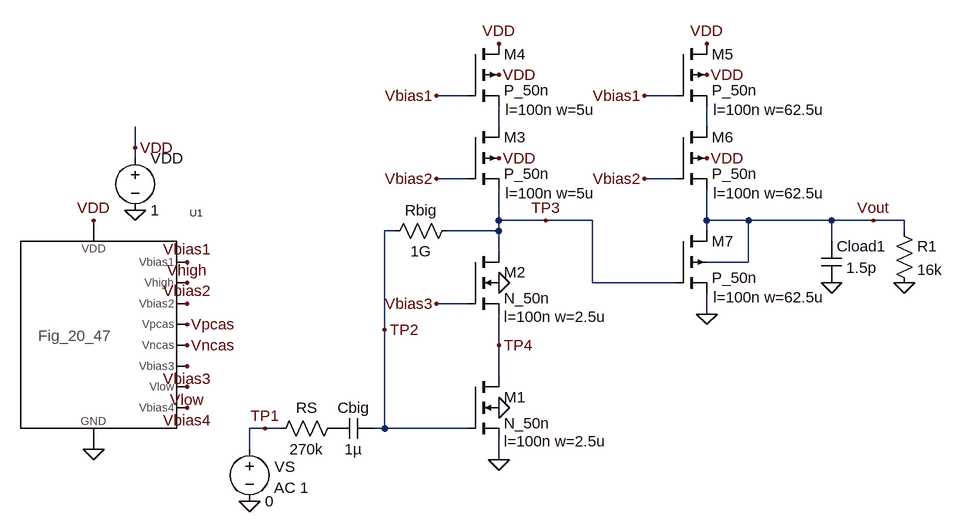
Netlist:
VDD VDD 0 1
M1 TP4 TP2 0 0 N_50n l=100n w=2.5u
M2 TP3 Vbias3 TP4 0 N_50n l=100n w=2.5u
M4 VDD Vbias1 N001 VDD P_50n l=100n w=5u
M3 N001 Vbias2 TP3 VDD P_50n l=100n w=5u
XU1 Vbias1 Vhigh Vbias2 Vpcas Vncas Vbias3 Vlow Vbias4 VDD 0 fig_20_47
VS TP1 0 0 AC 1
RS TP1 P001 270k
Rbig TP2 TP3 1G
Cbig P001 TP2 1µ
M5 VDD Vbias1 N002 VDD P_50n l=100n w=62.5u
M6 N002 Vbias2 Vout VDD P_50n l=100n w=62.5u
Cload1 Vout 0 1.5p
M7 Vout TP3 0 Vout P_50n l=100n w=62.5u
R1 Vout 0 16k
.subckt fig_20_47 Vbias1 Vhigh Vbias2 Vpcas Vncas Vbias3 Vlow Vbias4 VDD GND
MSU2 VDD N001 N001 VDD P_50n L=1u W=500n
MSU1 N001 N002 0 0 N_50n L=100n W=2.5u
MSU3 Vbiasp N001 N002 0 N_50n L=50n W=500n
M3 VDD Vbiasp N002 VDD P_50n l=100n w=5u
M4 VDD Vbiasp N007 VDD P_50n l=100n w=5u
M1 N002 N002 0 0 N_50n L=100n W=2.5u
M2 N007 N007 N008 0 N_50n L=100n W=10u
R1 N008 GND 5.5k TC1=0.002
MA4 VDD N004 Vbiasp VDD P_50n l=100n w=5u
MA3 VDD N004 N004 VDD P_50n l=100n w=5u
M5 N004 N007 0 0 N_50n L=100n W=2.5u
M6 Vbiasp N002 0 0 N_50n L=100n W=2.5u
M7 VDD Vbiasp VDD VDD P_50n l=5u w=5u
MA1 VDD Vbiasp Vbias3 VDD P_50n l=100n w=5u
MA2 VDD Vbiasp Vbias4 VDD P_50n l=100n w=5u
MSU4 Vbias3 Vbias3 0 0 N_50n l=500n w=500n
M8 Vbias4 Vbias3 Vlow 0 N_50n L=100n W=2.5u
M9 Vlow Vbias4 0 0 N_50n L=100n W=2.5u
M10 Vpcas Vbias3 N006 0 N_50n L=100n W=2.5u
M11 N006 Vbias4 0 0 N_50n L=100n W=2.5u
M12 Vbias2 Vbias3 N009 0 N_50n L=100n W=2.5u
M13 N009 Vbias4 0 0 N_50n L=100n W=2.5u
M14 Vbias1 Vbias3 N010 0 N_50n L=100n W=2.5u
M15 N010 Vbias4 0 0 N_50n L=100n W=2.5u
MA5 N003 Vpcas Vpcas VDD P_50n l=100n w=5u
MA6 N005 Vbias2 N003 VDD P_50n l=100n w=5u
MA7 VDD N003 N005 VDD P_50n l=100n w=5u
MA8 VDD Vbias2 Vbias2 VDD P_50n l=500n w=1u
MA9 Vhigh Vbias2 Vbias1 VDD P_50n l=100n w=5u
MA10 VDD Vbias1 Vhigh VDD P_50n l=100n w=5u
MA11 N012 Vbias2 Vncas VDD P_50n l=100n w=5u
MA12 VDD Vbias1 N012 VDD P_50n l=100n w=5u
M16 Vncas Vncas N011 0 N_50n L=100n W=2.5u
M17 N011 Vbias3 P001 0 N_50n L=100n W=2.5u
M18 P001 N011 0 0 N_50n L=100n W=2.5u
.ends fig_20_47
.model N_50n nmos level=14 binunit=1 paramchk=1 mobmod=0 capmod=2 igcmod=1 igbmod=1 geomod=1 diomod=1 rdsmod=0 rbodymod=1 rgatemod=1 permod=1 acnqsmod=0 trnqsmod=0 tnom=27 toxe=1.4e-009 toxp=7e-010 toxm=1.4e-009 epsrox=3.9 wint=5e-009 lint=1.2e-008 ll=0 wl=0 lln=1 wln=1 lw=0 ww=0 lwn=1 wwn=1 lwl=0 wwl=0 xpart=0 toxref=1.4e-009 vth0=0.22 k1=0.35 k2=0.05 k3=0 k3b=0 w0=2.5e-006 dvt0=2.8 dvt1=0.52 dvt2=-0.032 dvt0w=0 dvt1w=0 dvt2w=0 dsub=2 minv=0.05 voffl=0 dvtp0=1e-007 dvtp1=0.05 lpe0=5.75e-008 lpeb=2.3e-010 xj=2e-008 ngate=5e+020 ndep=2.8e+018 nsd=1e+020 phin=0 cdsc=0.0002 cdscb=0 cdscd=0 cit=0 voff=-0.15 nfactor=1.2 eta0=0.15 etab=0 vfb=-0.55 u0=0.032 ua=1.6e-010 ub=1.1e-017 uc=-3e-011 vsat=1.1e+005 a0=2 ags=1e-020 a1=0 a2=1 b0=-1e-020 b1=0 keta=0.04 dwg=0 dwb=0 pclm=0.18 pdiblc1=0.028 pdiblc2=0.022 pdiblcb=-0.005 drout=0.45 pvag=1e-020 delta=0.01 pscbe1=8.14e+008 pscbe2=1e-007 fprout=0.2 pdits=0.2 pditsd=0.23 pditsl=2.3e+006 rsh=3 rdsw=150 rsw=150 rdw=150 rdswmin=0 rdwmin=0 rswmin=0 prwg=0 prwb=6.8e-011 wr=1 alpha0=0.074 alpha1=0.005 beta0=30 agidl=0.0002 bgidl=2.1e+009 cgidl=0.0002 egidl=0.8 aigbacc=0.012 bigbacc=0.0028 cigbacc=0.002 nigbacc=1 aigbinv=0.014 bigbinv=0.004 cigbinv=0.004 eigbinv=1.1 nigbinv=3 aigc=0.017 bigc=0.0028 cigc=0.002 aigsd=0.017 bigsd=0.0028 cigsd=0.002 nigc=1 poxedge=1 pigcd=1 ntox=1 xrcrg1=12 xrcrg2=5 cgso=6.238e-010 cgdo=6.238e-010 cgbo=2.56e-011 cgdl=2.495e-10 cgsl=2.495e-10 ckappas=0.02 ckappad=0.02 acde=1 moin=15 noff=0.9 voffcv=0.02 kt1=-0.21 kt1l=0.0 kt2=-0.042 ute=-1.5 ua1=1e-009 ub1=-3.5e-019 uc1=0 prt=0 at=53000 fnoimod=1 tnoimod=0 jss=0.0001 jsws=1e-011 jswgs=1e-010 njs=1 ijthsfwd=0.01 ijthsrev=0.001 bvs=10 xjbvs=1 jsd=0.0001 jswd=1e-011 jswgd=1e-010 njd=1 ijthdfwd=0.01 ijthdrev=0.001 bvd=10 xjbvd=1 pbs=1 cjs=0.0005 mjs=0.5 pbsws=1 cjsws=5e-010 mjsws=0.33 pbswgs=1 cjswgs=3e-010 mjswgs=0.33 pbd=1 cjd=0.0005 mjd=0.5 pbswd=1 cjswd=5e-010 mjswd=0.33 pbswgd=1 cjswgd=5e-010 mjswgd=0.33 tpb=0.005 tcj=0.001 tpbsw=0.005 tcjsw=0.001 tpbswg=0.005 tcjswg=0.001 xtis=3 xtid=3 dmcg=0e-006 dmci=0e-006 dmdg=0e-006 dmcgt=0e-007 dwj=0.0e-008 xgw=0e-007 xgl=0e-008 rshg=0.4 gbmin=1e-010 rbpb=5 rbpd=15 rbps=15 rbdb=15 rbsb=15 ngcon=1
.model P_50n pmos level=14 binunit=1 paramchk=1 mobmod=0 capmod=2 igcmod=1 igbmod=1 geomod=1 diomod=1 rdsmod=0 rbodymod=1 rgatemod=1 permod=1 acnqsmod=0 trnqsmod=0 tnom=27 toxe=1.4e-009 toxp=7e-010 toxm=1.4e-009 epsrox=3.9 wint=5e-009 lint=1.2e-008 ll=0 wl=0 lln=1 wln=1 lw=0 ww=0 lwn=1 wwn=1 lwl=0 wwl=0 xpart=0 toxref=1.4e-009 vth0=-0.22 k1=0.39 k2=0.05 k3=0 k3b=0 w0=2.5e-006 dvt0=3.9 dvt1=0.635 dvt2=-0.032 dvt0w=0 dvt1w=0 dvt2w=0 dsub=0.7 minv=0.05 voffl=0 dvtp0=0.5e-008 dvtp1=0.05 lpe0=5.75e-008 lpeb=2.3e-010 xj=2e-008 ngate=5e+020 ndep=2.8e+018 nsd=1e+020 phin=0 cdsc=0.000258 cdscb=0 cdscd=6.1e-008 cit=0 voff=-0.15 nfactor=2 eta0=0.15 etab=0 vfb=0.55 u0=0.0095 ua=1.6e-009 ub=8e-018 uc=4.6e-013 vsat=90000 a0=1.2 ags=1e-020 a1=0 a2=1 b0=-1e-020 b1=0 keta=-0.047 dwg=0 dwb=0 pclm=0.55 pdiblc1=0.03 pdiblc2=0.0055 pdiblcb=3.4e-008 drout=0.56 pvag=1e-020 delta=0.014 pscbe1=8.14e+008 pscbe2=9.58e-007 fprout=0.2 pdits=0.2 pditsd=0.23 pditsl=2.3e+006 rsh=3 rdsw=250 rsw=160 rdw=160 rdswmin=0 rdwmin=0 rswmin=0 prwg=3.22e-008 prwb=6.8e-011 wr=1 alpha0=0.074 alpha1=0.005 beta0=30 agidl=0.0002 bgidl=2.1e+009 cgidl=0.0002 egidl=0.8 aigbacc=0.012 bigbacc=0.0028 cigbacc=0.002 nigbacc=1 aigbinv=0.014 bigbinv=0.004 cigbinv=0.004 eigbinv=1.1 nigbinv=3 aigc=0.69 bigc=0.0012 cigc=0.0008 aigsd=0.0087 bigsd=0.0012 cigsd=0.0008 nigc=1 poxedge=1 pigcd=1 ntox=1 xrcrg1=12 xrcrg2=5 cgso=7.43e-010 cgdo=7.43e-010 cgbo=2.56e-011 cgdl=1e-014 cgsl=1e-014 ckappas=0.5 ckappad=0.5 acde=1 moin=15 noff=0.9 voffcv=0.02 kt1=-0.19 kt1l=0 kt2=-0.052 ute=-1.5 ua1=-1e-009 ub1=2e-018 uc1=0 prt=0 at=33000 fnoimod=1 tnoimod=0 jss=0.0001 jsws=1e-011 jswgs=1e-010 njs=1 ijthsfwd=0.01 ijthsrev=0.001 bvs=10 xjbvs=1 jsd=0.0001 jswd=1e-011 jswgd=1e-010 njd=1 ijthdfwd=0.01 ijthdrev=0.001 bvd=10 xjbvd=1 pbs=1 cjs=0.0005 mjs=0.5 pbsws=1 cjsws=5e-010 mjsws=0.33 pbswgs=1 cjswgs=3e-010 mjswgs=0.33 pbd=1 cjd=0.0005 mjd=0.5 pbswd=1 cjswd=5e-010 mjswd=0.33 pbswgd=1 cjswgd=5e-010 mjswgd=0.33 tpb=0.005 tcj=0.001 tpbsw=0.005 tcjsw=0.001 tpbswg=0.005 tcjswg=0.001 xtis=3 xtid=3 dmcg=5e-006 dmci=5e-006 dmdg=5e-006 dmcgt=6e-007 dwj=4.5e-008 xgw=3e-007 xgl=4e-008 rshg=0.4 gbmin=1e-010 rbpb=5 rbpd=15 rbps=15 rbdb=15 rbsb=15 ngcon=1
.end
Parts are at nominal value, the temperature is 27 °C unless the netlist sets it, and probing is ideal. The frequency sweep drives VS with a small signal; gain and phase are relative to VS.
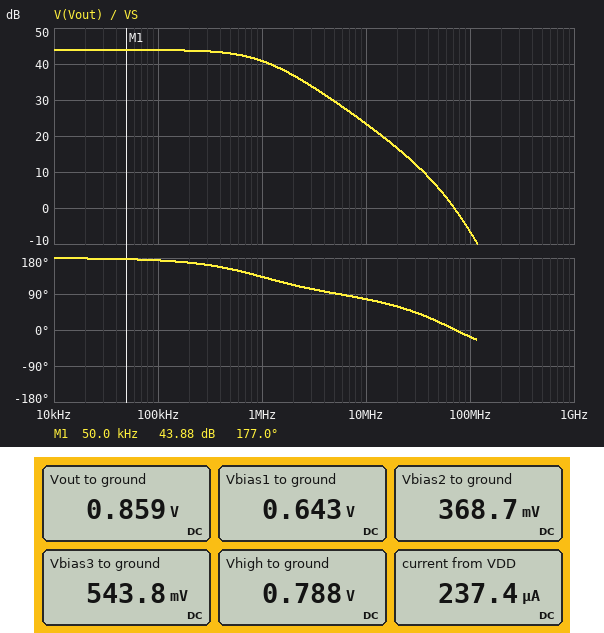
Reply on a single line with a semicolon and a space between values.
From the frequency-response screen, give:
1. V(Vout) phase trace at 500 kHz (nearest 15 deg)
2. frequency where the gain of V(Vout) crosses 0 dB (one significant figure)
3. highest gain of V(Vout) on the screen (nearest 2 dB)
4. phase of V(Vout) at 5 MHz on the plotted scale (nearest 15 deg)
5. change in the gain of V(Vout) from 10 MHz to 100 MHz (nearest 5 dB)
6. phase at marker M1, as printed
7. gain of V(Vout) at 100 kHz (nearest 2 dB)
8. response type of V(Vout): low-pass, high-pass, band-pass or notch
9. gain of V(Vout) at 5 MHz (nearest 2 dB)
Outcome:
150 deg; 70 MHz; 44 dB; 90 deg; -30 dB; 177.0 deg; 44 dB; low-pass; 30 dB
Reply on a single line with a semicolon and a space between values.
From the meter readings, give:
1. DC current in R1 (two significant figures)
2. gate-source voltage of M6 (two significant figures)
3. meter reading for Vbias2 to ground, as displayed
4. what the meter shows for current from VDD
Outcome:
54 µA; -490 mV; 368.7 mV; 237.4 µA
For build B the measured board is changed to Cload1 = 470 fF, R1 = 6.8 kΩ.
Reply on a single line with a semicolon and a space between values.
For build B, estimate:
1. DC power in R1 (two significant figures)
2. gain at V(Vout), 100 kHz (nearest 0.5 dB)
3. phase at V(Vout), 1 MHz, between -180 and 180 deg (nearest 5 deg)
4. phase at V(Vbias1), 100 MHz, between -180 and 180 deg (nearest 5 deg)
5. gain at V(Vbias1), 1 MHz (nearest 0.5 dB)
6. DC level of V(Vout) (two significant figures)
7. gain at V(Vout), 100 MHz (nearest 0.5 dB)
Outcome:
88 µW; 40.5 dB; 130 deg; 30 deg; -27.5 dB; 770 mV; -15.0 dB
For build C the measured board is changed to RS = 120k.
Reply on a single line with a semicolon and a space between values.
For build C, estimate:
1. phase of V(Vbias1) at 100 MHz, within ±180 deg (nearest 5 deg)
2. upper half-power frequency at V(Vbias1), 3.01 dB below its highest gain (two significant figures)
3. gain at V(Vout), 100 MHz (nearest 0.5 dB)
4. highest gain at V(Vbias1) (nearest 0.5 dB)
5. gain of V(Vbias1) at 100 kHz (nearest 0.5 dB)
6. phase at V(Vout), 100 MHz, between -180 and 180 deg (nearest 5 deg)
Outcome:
60 deg; 61 MHz; -3.0 dB; -17.0 dB; -37.0 dB; 5 deg
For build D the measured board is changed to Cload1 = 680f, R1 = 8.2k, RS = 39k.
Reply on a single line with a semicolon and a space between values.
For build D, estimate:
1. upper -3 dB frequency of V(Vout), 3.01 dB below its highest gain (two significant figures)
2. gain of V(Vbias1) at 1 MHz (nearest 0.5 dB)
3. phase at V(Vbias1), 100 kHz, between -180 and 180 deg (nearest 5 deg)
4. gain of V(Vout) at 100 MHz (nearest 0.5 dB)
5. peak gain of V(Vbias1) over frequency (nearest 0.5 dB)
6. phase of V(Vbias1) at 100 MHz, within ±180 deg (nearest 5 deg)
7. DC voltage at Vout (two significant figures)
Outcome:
950 kHz; -22.5 dB; -65 deg; -6.0 dB; -19.5 dB; 75 deg; 810 mV
